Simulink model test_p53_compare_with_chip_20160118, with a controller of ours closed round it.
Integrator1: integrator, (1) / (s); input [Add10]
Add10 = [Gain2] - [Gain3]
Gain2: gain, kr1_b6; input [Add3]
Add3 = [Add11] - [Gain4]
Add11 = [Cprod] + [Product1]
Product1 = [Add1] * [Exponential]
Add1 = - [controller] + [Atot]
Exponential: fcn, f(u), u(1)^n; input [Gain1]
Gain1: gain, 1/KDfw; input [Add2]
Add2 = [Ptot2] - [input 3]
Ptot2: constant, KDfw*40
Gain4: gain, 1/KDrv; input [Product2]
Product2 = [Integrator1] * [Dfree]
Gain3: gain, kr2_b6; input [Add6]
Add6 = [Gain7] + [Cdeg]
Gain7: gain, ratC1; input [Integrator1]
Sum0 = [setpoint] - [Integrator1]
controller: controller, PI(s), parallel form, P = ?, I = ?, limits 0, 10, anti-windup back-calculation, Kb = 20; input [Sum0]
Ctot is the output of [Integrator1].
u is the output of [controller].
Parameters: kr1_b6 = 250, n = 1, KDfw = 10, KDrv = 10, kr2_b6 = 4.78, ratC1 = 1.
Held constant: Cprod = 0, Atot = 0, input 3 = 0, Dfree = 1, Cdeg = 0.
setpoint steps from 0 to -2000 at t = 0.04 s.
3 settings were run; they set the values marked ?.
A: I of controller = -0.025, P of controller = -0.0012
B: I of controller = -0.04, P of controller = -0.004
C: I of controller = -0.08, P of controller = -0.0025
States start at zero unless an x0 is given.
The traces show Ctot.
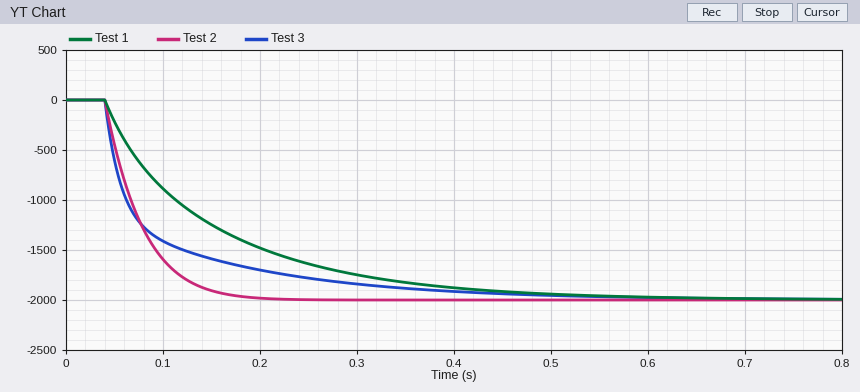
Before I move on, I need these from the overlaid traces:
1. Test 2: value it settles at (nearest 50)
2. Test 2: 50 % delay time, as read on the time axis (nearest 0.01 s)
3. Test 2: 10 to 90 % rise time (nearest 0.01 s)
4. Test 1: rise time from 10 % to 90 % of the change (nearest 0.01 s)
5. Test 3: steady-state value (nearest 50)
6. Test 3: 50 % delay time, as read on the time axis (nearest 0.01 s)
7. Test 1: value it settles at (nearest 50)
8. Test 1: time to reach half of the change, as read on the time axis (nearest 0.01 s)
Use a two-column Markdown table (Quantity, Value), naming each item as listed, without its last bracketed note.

| Quantity | Value |
|---|---|
| Test 2: value it settles at | -2000 |
| Test 2: 50 % delay time, as read on the time axis | 0.07 s |
| Test 2: 10 to 90 % rise time | 0.08 s |
| Test 1: rise time from 10 % to 90 % of the change | 0.28 s |
| Test 3: steady-state value | -2000 |
| Test 3: 50 % delay time, as read on the time axis | 0.06 s |
| Test 1: value it settles at | -2000 |
| Test 1: time to reach half of the change, as read on the time axis | 0.11 s |
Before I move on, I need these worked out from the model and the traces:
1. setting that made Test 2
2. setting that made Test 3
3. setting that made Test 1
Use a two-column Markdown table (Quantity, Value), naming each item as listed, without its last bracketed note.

| Quantity | Value |
|---|---|
| setting that made Test 2 | C |
| setting that made Test 3 | B |
| setting that made Test 1 | A |
